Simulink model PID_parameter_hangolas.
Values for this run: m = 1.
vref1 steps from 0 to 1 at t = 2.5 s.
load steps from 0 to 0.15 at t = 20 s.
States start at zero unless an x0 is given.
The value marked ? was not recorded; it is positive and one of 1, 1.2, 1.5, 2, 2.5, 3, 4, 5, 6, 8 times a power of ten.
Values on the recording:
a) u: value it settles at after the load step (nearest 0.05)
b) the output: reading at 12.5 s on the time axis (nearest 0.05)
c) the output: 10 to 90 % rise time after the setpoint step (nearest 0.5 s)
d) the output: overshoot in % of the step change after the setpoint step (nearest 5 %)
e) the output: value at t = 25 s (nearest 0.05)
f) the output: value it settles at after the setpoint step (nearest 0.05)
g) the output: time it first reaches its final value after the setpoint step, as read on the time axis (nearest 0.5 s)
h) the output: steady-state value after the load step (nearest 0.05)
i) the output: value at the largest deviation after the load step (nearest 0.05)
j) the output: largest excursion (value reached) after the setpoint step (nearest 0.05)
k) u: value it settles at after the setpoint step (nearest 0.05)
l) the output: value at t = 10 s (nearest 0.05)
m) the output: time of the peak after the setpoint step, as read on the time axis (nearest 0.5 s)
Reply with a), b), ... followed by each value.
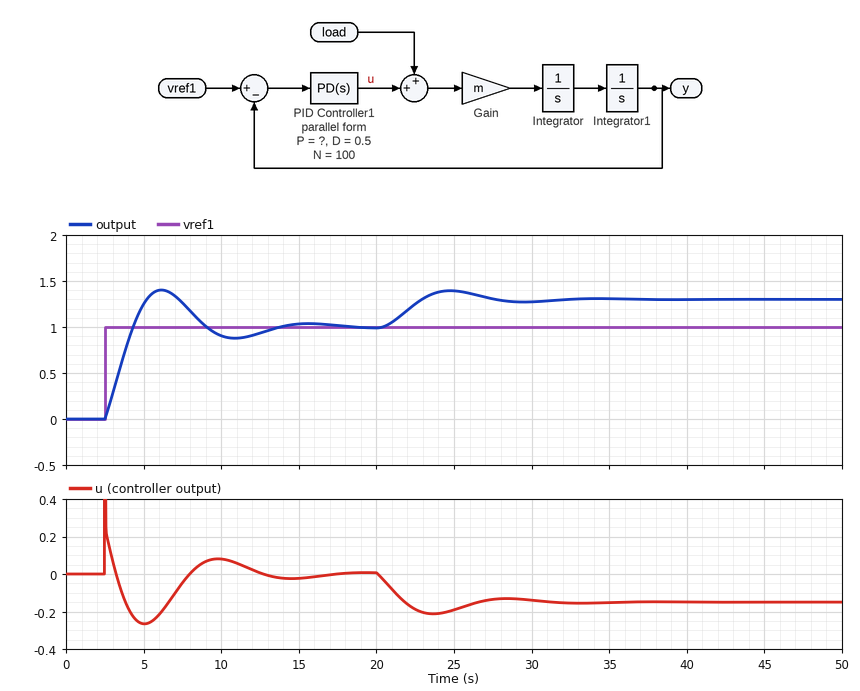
a) -0.15
b) 0.95
c) 1.5 s
d) 40 %
e) 1.40
f) 1.00
g) 4.5 s
h) 1.30
i) 1.40
j) 1.40
k) 0.00
l) 0.90
m) 6.0 s
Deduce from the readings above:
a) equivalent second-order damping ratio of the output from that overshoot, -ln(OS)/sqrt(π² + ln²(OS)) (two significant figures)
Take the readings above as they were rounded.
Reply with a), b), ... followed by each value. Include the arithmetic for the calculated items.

a) ln(0.4) = -0.916; 0.916 / sqrt(9.870 + 0.840) = 0.28
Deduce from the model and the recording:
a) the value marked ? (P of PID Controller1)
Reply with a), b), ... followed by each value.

a) 0.5
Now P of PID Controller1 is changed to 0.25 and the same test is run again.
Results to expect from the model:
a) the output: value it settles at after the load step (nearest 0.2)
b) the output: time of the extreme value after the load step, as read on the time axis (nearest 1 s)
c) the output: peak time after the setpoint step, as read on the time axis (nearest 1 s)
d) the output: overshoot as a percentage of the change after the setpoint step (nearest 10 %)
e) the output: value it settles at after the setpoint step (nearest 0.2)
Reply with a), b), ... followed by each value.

a) 1.6
b) 27 s
c) 7 s
d) 30 %
e) 1.0
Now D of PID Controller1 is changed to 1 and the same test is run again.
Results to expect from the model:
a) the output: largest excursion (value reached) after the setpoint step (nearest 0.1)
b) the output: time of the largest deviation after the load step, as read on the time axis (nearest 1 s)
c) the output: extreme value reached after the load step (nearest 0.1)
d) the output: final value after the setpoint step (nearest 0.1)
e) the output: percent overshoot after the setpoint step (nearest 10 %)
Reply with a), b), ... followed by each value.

a) 1.2
b) 26 s
c) 1.3
d) 1.0
e) 20 %
